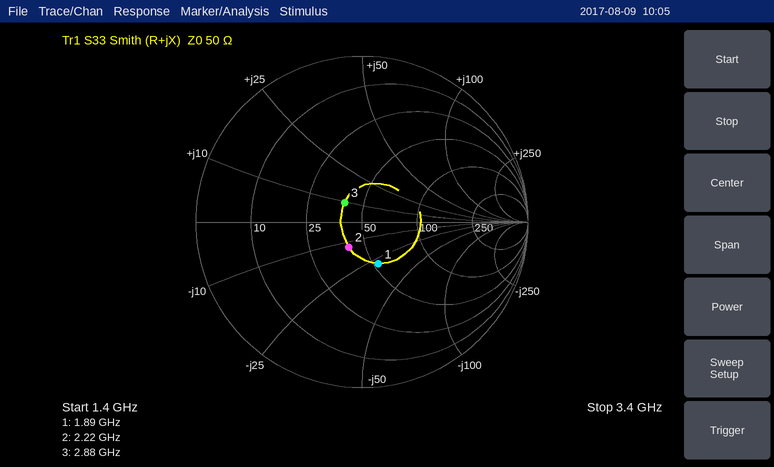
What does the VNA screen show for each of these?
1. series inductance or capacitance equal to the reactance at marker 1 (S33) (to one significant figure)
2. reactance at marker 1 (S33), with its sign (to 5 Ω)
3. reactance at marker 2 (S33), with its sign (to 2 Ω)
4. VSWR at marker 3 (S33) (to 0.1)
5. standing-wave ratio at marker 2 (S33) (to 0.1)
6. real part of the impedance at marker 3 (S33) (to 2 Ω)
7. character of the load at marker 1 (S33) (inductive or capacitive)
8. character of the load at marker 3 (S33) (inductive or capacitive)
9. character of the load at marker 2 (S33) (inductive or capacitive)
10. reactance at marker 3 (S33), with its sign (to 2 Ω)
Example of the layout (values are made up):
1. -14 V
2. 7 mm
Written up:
1. 3 pF
2. -30 Ω
3. -12 Ω
4. 1.4
5. 1.4
6. 40 Ω
7. capacitive
8. inductive
9. capacitive
10. +10 Ω
